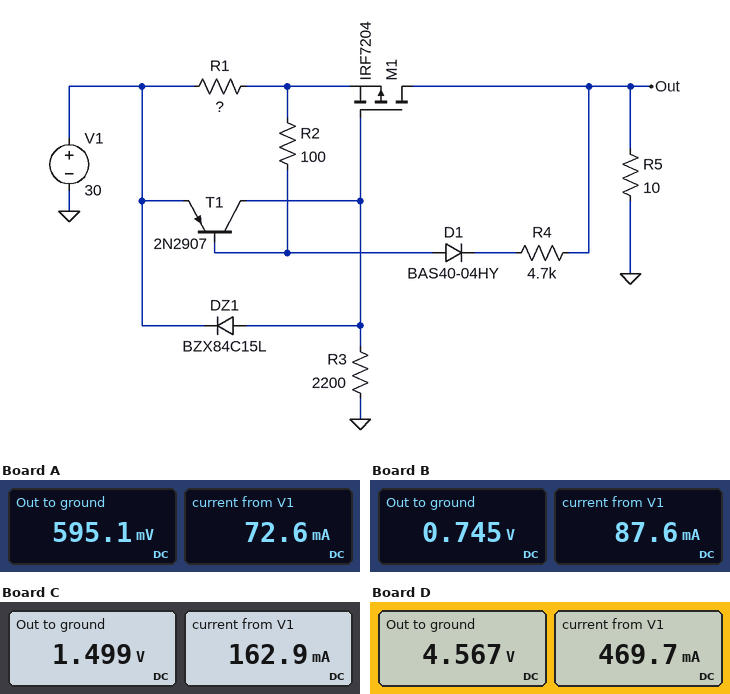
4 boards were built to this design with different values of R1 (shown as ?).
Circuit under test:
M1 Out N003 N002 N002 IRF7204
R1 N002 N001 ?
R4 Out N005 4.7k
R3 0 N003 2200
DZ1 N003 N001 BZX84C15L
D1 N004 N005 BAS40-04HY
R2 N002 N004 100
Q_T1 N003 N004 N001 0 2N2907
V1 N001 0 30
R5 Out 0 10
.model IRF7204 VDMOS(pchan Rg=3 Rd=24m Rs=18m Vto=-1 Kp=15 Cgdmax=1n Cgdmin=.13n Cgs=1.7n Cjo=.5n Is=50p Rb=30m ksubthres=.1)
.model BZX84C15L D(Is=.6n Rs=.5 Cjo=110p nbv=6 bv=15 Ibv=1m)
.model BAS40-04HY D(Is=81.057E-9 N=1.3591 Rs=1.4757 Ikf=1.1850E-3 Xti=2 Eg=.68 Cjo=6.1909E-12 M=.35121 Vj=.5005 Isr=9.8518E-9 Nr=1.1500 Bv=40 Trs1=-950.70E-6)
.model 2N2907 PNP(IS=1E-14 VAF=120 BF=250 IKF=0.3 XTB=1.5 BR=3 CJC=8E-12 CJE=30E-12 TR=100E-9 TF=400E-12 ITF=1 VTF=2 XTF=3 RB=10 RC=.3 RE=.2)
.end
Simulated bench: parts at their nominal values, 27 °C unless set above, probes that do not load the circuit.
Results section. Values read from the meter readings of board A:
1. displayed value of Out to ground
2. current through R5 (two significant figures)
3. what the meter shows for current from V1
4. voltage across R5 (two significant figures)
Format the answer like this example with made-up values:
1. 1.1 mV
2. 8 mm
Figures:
1. 595.1 mV
2. 60 mA
3. 72.6 mA
4. 600 mV
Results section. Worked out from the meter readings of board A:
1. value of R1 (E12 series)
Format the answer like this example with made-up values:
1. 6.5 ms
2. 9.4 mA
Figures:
1. 2.2 Ω
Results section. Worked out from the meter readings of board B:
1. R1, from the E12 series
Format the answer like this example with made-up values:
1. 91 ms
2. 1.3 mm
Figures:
1. 1.8 Ω
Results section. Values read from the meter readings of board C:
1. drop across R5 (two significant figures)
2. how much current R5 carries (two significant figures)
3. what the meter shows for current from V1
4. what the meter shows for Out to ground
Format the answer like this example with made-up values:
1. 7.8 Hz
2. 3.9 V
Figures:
1. 1.5 V
2. 150 mA
3. 162.9 mA
4. 1.499 V
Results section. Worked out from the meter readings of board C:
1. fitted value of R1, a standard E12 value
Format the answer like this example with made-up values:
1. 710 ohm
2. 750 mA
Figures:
1. 1 Ω
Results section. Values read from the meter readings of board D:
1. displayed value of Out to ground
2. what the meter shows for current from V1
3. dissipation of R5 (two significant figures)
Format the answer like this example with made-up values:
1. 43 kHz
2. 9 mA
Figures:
1. 4.567 V
2. 469.7 mA
3. 2.1 W
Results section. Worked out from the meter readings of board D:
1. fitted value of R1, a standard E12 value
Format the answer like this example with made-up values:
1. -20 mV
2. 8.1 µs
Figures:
1. 0.47 Ω
